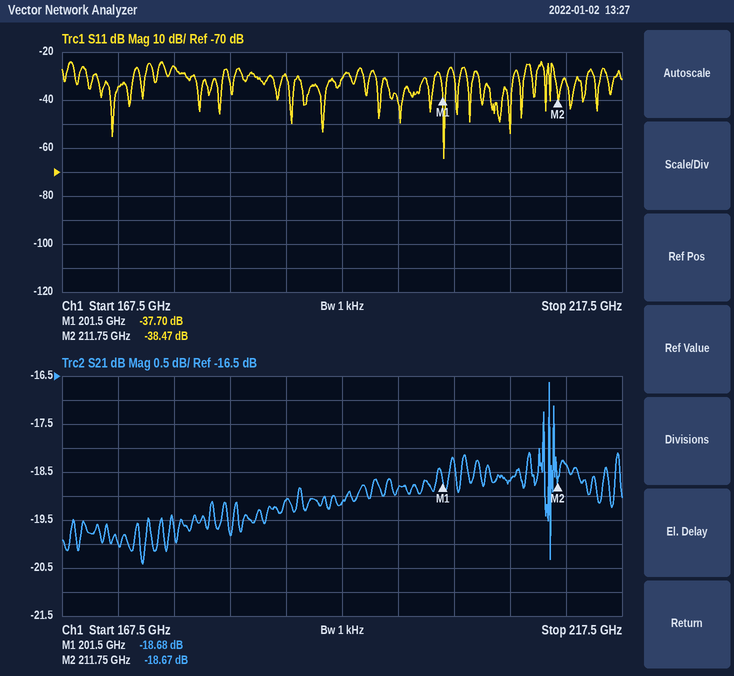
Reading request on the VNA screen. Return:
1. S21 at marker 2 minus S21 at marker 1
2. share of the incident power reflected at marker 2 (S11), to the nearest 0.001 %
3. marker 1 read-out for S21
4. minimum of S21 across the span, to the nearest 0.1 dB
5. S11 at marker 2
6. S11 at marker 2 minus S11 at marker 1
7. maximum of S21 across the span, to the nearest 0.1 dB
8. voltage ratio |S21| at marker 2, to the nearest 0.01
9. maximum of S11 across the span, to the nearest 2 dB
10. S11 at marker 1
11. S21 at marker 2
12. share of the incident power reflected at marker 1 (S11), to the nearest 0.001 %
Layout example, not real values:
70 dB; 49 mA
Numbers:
0.01 dB; 0.014 %; -18.68 dB; -20.4 dB; -38.47 dB; -0.77 dB; -16.6 dB; 0.12; -24 dB; -37.70 dB; -18.67 dB; 0.017 %
